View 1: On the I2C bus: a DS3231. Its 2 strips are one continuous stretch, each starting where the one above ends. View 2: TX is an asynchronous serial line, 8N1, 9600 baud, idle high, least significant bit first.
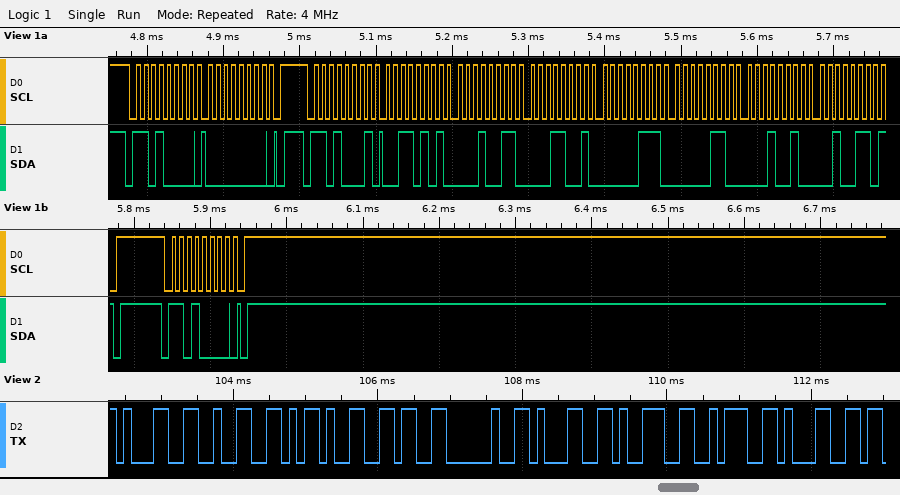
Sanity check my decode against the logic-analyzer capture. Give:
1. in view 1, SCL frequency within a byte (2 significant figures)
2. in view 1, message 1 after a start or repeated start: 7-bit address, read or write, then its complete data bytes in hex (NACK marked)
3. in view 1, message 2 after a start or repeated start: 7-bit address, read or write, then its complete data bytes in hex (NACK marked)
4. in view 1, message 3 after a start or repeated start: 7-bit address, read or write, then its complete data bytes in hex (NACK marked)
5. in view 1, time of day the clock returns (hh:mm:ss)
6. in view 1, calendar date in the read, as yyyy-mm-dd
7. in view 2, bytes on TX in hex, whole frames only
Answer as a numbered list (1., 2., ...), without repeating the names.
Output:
1. 100 kHz
2. 0x68 write: 00
3. 0x68 read: 35 13 19 07 06 12 26 NACK
4. 0x68 write
5. 19:13:35
6. 2026-12-06
7. 31 32 2D 36 20 31 39 3A 31
